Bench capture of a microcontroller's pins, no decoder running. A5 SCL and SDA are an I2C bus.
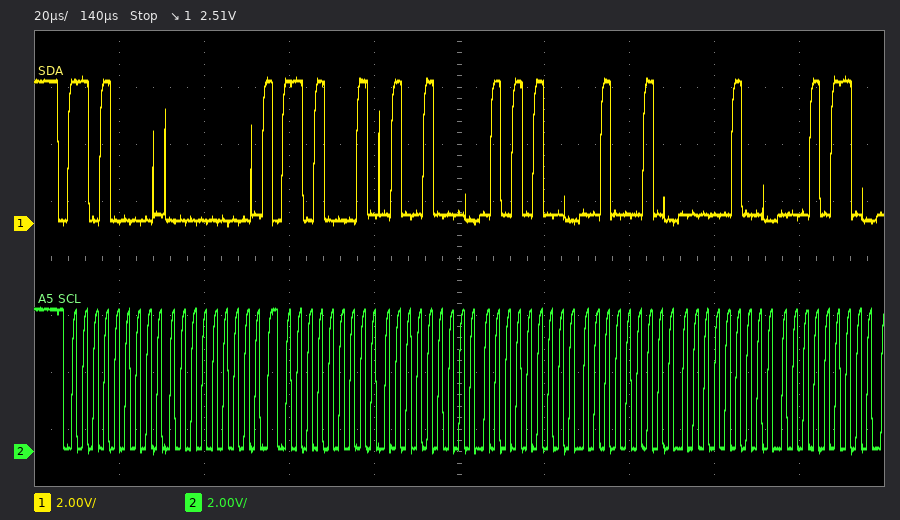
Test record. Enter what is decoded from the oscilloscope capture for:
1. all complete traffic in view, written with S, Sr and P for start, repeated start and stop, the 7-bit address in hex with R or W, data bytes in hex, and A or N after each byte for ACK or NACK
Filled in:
S 68W A 00 A Sr 68R A 48 A 54 A 22 A 04 A 16 A
